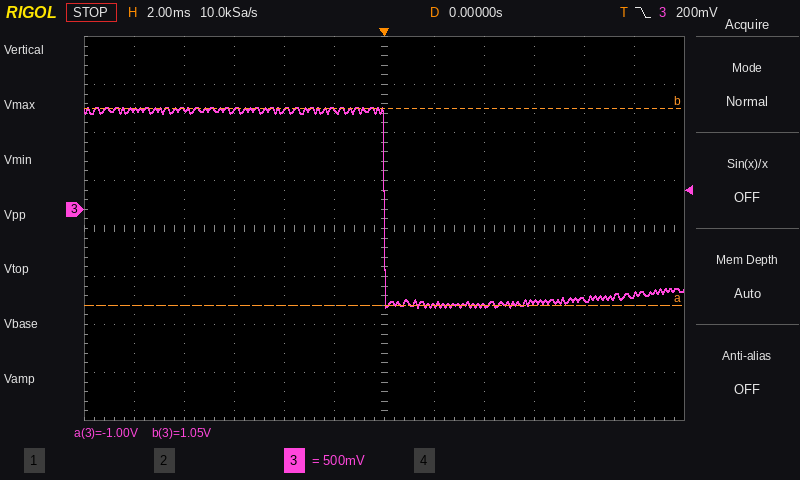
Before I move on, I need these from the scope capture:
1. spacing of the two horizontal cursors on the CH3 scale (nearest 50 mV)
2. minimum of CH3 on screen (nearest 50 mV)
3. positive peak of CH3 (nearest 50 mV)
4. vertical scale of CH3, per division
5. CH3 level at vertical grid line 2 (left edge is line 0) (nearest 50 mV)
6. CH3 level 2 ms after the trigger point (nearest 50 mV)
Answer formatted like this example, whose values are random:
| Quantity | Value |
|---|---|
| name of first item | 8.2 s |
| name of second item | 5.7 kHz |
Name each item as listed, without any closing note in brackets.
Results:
| Quantity | Value |
|---|---|
| spacing of the two horizontal cursors on the CH3 scale | 2.05 V |
| minimum of CH3 on screen | -1.00 V |
| positive peak of CH3 | 1.05 V |
| vertical scale of CH3, per division | 500 mV |
| CH3 level at vertical grid line 2 (left edge is line 0) | 1.05 V |
| CH3 level 2 ms after the trigger point | -1.00 V |
